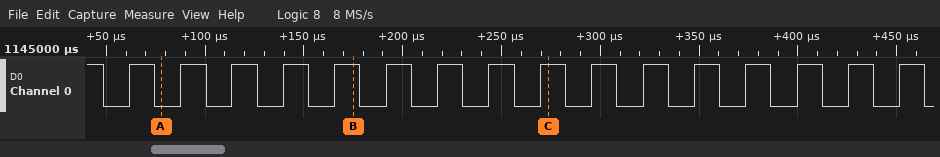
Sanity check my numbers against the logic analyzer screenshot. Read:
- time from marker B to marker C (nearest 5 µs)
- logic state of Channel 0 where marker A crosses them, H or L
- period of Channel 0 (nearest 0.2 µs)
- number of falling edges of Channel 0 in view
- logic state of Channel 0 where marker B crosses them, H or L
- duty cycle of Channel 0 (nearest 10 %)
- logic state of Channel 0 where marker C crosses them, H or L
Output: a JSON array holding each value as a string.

["100 µs", "Channel 0=L", "26 µs", "17", "Channel 0=H", "50 %", "Channel 0=H"]
